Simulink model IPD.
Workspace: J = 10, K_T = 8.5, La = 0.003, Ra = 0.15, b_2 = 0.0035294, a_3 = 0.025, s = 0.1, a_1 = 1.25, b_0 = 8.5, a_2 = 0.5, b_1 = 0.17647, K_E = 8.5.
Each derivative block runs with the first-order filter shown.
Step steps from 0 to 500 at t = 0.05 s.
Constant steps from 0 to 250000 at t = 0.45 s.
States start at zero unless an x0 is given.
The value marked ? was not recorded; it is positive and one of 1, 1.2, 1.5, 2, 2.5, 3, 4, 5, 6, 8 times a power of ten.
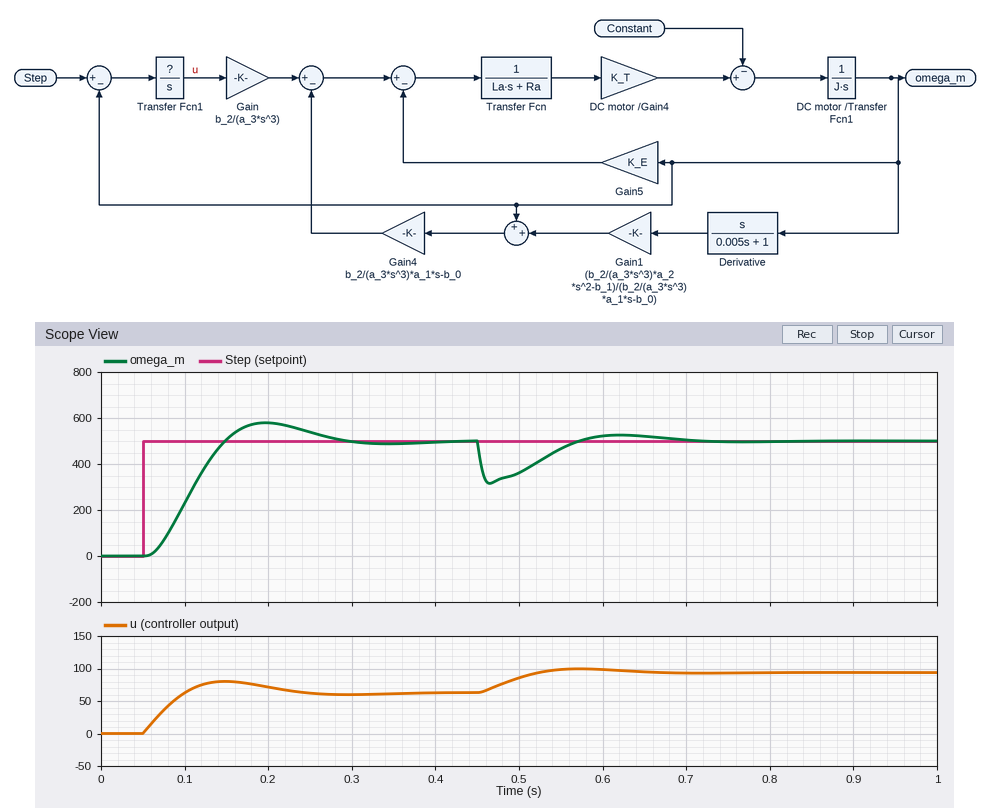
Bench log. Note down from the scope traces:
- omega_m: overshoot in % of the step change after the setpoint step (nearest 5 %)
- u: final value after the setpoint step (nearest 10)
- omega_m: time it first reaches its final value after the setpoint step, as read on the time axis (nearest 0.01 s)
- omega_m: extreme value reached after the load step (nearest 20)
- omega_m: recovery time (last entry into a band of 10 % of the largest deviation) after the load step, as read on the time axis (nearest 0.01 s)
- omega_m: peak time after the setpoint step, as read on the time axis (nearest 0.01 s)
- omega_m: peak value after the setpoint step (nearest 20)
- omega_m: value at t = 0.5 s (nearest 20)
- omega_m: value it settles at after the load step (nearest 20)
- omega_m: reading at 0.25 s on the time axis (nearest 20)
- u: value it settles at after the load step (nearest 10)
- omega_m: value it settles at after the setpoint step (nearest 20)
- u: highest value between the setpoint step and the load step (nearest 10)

15 %
60
0.15 s
320
0.66 s
0.20 s
580
360
500
540
90
500
80
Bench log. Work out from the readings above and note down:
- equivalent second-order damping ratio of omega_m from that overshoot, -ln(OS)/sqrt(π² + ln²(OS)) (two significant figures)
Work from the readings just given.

0.52
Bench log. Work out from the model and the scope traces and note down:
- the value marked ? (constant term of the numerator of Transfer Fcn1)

3
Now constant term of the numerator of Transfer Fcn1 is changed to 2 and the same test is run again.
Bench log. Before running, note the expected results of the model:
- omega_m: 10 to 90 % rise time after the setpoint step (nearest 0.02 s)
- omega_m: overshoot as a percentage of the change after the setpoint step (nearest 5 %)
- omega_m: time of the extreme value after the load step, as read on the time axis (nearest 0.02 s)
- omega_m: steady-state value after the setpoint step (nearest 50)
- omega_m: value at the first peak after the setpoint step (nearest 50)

0.10 s
10 %
0.46 s
500
550
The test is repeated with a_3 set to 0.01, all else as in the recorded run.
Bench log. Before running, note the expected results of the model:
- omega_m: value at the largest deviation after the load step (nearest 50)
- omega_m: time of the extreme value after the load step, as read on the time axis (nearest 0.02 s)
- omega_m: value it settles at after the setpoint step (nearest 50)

400
0.46 s
500
